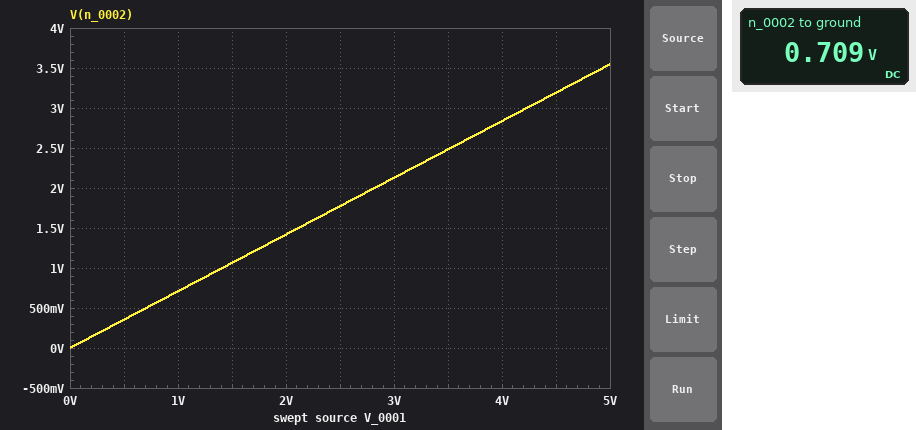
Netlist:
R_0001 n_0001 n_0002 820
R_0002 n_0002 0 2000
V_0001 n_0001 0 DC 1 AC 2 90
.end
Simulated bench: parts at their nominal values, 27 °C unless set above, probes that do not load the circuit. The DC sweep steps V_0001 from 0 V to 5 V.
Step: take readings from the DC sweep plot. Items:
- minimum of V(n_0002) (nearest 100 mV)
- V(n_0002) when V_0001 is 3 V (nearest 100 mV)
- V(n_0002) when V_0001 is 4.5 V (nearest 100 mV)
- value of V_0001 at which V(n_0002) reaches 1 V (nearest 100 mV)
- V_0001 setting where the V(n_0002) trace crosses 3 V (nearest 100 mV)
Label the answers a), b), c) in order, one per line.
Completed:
a) 0 V
b) 2.1 V
c) 3.2 V
d) 1.4 V
e) 4.2 V
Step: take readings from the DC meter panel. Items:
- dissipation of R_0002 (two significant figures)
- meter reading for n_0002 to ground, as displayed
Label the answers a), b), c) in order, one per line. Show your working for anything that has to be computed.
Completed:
a) (709 mV)^2 / 2 kΩ = 250 µW
b) 0.709 V
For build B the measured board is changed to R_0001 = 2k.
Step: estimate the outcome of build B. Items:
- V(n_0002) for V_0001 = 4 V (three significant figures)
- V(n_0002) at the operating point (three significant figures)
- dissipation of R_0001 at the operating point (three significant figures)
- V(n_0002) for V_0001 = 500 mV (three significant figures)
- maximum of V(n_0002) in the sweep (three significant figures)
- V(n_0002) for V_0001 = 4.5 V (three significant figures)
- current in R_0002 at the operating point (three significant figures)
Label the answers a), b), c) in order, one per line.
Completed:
a) 2.00 V
b) 500 mV
c) 125 µW
d) 250 mV
e) 2.50 V
f) 2.25 V
g) 250 µA
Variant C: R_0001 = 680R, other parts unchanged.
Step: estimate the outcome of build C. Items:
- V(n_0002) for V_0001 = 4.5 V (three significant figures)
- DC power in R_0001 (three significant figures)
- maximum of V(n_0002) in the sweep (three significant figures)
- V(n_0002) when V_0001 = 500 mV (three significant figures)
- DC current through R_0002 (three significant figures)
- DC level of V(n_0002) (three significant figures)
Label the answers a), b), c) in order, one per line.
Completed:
a) 3.36 V
b) 94.7 µW
c) 3.73 V
d) 373 mV
e) 373 µA
f) 746 mV
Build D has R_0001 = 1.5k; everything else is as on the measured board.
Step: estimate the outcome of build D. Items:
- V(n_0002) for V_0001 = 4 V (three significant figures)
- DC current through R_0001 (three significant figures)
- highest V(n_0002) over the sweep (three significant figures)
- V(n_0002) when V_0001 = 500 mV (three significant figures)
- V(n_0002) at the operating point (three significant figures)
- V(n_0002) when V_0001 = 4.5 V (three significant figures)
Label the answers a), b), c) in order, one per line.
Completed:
a) 2.29 V
b) 286 µA
c) 2.86 V
d) 286 mV
e) 571 mV
f) 2.57 V
